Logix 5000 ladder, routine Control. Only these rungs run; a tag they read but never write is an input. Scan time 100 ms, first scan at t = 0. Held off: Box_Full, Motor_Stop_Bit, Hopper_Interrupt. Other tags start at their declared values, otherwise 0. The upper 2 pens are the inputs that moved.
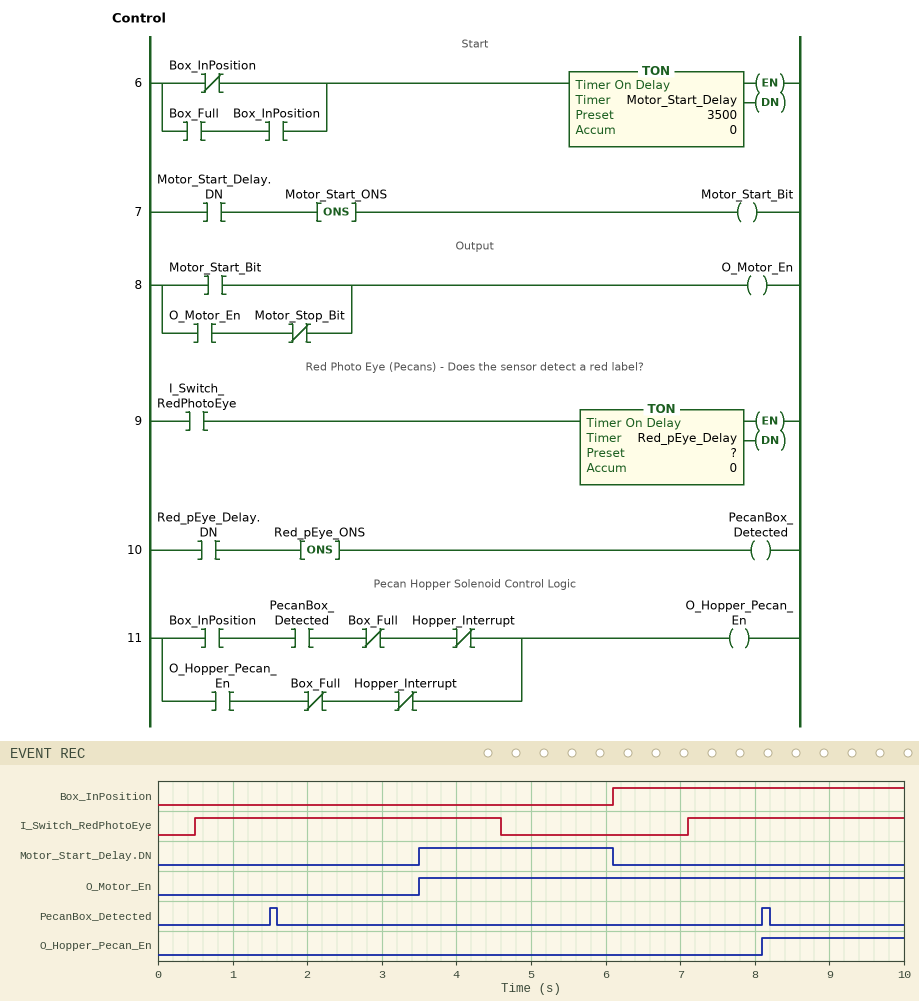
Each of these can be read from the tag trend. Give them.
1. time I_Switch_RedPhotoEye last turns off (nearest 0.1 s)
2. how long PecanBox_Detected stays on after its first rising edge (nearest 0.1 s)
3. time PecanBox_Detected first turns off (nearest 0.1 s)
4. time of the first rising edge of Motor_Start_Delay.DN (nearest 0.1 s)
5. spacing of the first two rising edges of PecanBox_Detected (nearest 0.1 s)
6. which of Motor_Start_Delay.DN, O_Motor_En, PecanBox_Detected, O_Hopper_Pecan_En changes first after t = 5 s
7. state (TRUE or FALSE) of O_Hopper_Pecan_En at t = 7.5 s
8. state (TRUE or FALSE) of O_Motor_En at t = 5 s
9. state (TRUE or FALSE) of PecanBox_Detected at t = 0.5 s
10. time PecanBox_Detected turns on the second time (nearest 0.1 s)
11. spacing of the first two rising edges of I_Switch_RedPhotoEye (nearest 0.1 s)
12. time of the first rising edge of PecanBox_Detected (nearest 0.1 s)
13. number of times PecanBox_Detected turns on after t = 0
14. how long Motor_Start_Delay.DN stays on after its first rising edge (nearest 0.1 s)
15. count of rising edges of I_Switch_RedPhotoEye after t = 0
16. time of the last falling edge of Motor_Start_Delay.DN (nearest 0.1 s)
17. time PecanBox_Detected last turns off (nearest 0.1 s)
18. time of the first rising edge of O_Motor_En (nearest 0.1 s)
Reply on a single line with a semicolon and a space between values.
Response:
4.6 s; 0.1 s; 1.6 s; 3.5 s; 6.6 s; Motor_Start_Delay.DN; FALSE; TRUE; FALSE; 8.1 s; 6.6 s; 1.5 s; 2; 2.6 s; 2; 6.1 s; 8.2 s; 3.5 s
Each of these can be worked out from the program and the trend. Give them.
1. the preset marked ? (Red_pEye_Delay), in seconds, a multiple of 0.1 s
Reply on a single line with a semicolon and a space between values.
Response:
1.0 s
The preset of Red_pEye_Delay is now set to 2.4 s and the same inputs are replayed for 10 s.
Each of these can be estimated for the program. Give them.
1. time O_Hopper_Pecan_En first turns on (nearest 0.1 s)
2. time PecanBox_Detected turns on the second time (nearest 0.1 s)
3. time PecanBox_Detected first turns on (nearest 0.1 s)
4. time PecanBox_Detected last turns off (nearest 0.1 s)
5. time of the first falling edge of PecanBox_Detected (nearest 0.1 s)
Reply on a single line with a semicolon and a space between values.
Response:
9.5 s; 9.5 s; 2.9 s; 9.6 s; 3.0 s
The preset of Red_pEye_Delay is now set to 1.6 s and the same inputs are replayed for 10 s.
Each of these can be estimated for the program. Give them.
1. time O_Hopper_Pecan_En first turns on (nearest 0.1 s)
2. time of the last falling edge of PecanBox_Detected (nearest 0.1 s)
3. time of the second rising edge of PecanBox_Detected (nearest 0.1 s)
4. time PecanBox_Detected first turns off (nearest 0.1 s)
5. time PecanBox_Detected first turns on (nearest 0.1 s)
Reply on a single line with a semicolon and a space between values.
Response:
8.7 s; 8.8 s; 8.7 s; 2.2 s; 2.1 s
